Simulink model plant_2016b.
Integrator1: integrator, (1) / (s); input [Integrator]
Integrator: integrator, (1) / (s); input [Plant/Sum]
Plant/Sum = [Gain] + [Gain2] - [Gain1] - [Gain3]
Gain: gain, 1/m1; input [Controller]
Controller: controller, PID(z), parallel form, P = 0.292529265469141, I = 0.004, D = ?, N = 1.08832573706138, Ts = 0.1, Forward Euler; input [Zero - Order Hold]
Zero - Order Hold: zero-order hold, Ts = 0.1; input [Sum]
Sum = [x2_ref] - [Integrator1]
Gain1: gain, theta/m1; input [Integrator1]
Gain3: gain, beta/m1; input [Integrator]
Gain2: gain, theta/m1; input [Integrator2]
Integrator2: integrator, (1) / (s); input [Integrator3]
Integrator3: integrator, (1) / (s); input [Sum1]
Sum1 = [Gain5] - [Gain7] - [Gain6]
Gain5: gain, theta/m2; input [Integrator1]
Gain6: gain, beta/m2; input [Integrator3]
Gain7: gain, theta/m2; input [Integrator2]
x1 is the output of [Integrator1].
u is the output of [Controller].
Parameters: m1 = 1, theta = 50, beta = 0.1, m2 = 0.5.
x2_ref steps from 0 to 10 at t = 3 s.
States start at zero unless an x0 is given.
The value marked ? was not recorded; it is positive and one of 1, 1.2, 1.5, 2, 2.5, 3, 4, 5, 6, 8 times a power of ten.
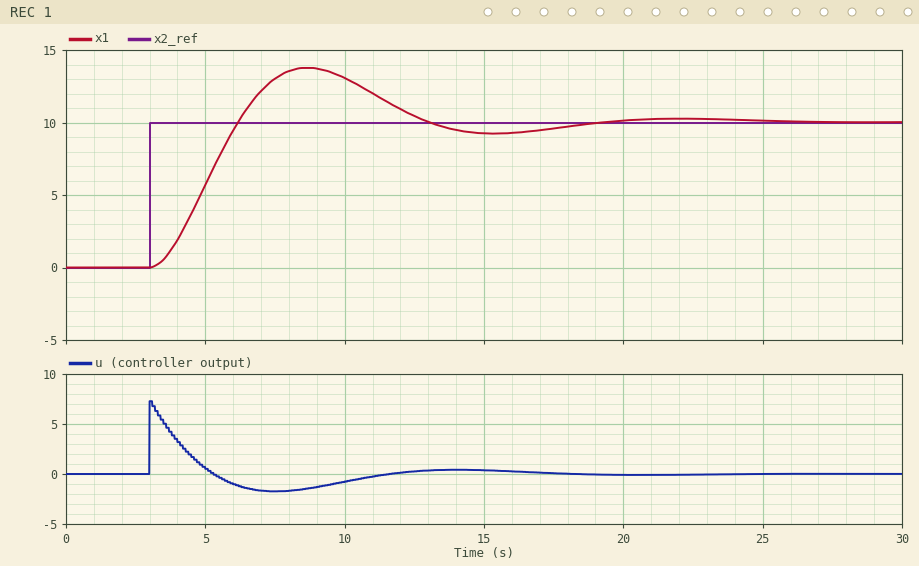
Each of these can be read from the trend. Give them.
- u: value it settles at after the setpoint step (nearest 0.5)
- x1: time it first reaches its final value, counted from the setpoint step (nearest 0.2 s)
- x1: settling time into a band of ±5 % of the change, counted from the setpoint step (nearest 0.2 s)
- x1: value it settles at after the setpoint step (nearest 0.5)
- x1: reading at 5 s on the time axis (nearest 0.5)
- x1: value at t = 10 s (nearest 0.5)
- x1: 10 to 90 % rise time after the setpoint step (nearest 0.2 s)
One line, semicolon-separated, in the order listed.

0.0; 3.2 s; 14.2 s; 10.0; 5.5; 13.0; 2.2 s
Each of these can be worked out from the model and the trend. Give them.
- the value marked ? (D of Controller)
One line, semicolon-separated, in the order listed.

0.4
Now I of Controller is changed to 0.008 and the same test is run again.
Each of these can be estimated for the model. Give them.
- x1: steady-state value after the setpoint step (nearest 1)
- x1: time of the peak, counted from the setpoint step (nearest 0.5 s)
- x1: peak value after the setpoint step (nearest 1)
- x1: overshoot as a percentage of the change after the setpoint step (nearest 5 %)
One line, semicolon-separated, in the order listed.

10; 6.0 s; 14; 40 %
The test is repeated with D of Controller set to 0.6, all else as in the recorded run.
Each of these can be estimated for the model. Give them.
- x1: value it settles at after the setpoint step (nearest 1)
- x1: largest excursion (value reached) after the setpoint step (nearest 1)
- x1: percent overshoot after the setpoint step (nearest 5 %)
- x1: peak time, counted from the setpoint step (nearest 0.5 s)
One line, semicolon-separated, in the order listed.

10; 13; 30 %; 5.0 s
